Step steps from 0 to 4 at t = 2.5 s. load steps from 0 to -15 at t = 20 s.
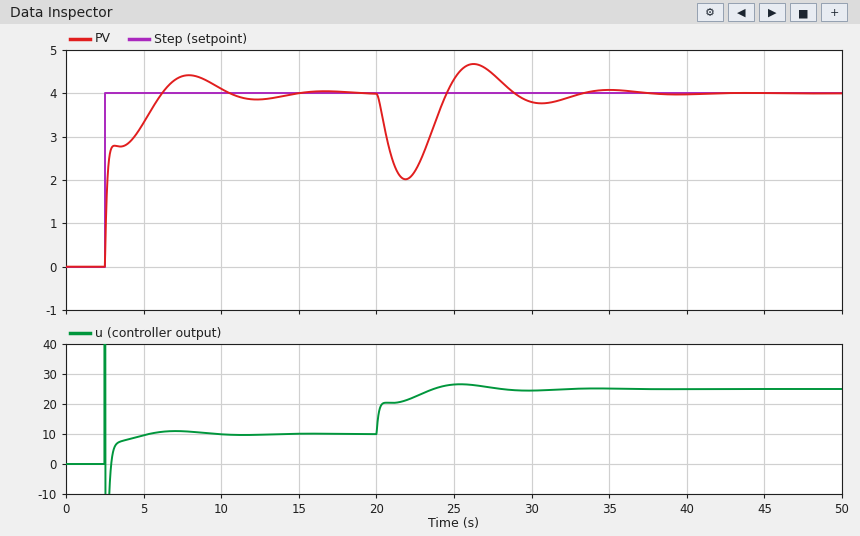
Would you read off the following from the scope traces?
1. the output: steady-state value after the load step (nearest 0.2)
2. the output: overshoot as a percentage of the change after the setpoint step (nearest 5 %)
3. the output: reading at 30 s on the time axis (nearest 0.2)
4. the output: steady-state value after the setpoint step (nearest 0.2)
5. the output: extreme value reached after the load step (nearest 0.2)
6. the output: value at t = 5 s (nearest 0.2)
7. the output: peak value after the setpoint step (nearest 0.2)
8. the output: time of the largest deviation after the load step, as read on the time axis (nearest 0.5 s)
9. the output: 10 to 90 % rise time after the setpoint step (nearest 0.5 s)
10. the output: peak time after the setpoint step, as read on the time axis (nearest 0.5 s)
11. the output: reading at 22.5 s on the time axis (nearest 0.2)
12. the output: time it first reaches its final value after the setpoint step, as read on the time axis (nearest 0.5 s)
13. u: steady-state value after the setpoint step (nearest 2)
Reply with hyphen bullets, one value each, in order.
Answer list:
- 4.0
- 10 %
- 3.8
- 4.0
- 2.0
- 3.4
- 4.4
- 22.0 s
- 3.0 s
- 8.0 s
- 2.2
- 6.0 s
- 10
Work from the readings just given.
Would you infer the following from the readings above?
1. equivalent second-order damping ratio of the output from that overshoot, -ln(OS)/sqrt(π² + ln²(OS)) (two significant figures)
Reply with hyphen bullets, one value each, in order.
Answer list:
- 0.59
